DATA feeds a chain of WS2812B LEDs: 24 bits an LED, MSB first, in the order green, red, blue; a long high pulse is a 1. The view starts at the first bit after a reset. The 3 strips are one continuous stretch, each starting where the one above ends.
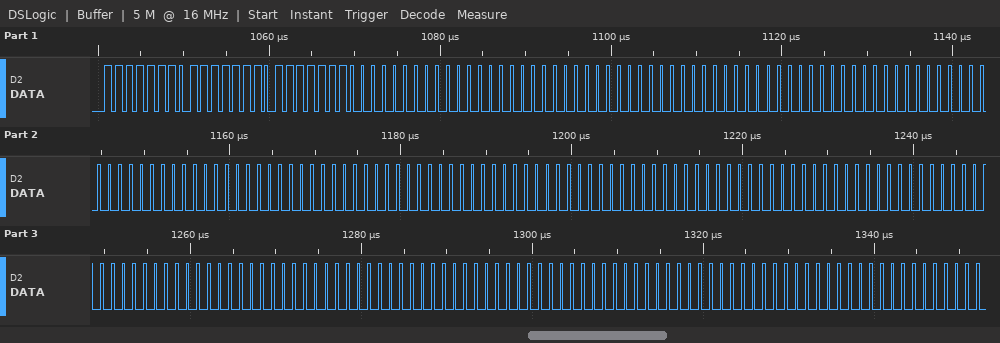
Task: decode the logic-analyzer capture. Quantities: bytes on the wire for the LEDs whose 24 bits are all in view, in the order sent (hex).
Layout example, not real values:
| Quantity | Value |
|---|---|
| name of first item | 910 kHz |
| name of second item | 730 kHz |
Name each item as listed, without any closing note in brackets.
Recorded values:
| Quantity | Value |
|---|---|
| bytes on the wire for the LEDs whose 24 bits are all in view, in the order sent | FE FE FE 00 00 00 00 00 00 00 00 00 00 00 00 00 00 00 00 00 00 00 00 00 00 00 00 00 00 00 |
